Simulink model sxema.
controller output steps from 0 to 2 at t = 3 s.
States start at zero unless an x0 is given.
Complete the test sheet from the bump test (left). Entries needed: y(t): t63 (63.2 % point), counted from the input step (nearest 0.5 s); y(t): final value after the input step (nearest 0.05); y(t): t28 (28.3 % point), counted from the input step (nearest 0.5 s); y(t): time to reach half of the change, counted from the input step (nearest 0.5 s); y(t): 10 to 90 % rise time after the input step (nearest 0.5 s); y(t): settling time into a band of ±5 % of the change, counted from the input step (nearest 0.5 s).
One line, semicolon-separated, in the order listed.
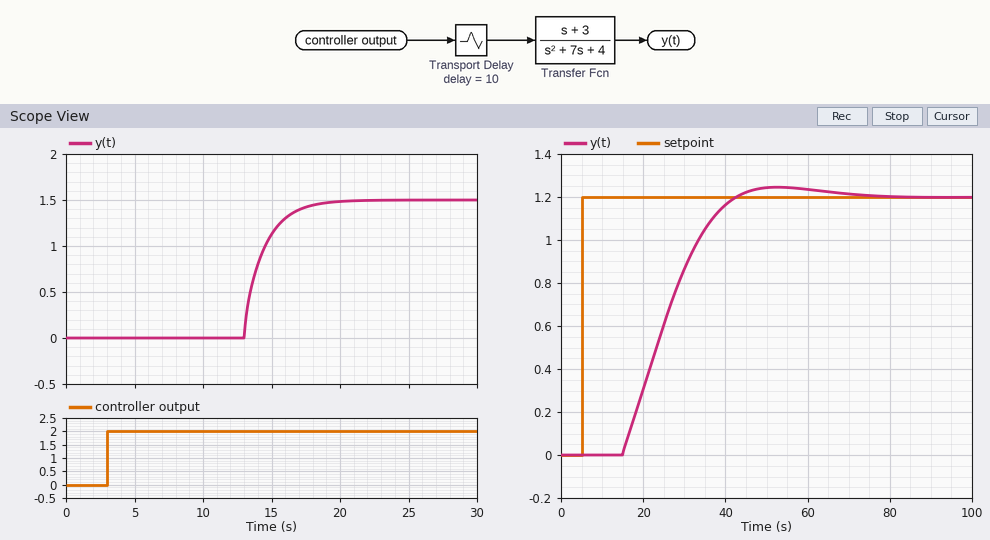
11.5 s; 1.50; 10.5 s; 11.0 s; 3.5 s; 14.5 s
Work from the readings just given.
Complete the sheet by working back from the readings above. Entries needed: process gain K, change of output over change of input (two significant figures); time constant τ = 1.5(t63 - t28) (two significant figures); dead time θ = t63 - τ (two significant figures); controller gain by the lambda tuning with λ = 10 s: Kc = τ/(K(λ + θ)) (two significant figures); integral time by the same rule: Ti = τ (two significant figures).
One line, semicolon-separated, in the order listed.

0.75; 1.5 s; 10 s; 0.10; 1.5 s
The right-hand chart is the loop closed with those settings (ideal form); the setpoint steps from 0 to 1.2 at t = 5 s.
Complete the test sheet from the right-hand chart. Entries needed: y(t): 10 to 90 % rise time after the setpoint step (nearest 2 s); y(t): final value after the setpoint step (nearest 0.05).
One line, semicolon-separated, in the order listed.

20 s; 1.20
